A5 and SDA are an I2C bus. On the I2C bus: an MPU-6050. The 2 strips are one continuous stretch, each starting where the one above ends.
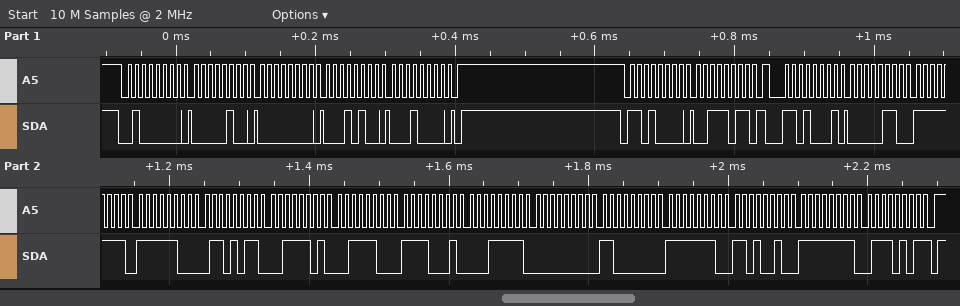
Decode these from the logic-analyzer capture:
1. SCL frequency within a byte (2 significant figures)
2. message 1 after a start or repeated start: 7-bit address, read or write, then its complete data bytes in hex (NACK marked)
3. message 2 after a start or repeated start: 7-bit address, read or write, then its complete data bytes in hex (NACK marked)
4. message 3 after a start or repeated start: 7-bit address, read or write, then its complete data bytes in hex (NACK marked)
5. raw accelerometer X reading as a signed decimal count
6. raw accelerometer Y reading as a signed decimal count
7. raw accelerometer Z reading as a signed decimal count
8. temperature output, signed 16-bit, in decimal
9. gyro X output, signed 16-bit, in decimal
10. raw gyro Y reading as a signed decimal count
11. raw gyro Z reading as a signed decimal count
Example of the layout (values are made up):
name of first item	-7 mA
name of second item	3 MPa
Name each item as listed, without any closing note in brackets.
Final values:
SCL frequency within a byte	100 kHz
message 1 after a start or repeated start: 7-bit address, read or write, then its complete data bytes in hex	0x20 write: 04 00 14 10
message 2 after a start or repeated start: 7-bit address, read or write, then its complete data bytes in hex	0x68 write: 3B
message 3 after a start or repeated start: 7-bit address, read or write, then its complete data bytes in hex	0x68 read: 06 FF FC 6B 3D 3C F1 1F 00 C0 FE D2 FF 75 NACK
raw accelerometer X reading as a signed decimal count	1791
raw accelerometer Y reading as a signed decimal count	-917
raw accelerometer Z reading as a signed decimal count	15676
temperature output, signed 16-bit, in decimal	-3809
gyro X output, signed 16-bit, in decimal	192
raw gyro Y reading as a signed decimal count	-302
raw gyro Z reading as a signed decimal count	-139
